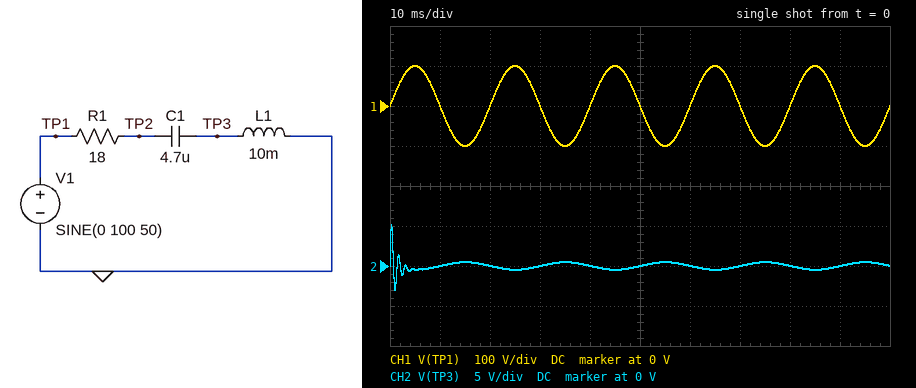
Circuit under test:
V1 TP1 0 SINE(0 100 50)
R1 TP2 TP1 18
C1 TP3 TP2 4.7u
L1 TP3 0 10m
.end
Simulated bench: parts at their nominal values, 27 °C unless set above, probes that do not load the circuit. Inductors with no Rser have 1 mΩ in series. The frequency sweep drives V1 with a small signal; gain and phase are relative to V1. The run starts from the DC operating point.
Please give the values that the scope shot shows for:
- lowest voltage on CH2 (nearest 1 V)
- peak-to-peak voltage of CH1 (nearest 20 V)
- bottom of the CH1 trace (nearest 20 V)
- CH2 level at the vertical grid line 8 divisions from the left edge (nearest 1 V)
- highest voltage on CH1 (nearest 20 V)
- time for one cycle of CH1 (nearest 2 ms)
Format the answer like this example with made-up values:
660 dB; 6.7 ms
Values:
-3 V; 200 V; -100 V; 0 V; 100 V; 20 ms
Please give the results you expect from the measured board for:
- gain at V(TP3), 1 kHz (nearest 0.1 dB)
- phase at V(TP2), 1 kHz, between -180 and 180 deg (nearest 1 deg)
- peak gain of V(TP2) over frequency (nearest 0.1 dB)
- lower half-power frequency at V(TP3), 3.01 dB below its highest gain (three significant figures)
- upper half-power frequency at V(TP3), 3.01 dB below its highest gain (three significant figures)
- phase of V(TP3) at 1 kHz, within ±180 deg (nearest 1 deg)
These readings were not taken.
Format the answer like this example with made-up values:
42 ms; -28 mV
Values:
5.3 dB; 32 deg; 0 dB; 642 Hz; 998 Hz; 32 deg
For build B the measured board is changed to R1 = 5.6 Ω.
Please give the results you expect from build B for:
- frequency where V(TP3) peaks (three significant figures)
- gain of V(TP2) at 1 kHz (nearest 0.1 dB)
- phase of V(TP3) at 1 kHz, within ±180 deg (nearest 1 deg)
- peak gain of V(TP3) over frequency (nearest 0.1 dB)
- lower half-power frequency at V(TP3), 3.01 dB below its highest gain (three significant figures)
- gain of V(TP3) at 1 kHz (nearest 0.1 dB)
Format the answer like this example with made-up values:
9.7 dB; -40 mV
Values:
737 Hz; -0.2 dB; 11 deg; 18.3 dB; 696 Hz; 6.6 dB
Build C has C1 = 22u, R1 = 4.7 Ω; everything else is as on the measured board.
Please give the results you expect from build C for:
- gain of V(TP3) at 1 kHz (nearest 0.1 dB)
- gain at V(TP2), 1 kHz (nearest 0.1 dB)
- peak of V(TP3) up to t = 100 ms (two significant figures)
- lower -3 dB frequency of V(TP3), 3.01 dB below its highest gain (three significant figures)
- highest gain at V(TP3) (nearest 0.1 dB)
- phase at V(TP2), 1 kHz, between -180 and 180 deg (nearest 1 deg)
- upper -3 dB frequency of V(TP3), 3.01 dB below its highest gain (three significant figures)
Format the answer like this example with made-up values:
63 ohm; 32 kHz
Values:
1.0 dB; 0 dB; 12 V; 310 Hz; 13.2 dB; 5 deg; 390 Hz
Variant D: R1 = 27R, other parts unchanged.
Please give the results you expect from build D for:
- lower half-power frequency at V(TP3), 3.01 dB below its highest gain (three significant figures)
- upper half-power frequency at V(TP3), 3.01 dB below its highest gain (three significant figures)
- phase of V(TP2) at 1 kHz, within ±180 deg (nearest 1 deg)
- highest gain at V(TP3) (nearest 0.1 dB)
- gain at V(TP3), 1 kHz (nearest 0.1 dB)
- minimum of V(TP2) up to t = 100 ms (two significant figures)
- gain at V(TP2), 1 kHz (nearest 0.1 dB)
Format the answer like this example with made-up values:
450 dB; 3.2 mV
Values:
623 Hz; 1.42 kHz; 43 deg; 5.0 dB; 4.0 dB; -100 V; -2.7 dB
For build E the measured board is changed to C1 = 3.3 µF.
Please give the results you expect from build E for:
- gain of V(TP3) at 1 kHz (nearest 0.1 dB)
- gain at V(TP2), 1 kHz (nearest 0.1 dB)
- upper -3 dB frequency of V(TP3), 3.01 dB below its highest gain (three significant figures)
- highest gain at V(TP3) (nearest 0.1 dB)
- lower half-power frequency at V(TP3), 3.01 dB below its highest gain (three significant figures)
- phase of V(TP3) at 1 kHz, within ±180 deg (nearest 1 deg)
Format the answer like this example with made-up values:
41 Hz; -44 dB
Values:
8.7 dB; -4.0 dB; 1.11 kHz; 9.8 dB; 778 Hz; 51 deg
